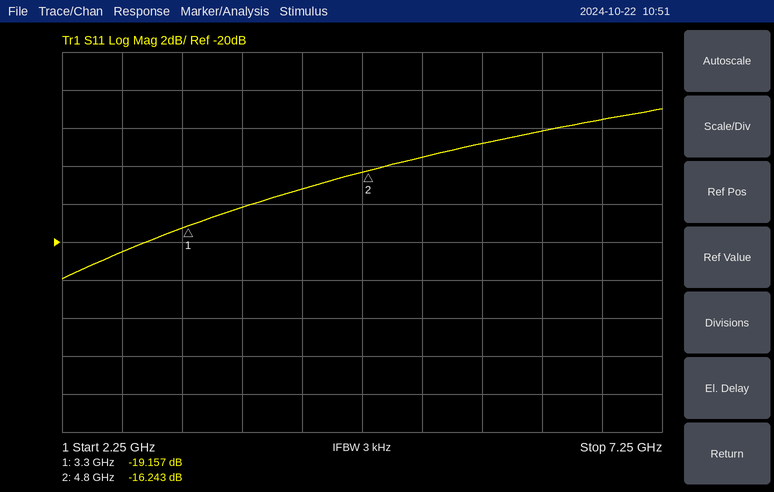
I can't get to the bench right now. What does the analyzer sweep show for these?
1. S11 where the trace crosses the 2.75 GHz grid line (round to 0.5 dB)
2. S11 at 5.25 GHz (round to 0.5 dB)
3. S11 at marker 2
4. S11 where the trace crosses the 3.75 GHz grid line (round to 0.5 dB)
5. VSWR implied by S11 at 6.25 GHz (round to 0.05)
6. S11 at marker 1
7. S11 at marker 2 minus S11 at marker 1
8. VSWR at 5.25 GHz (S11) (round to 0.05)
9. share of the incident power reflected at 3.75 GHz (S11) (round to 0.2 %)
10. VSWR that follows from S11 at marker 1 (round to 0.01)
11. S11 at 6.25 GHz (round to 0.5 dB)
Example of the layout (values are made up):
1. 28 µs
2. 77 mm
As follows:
1. -20.5 dB
2. -15.5 dB
3. -16.243 dB
4. -18.0 dB
5. 1.50
6. -19.157 dB
7. 2.914 dB
8. 1.40
9. 1.6 %
10. 1.25
11. -14.0 dB
